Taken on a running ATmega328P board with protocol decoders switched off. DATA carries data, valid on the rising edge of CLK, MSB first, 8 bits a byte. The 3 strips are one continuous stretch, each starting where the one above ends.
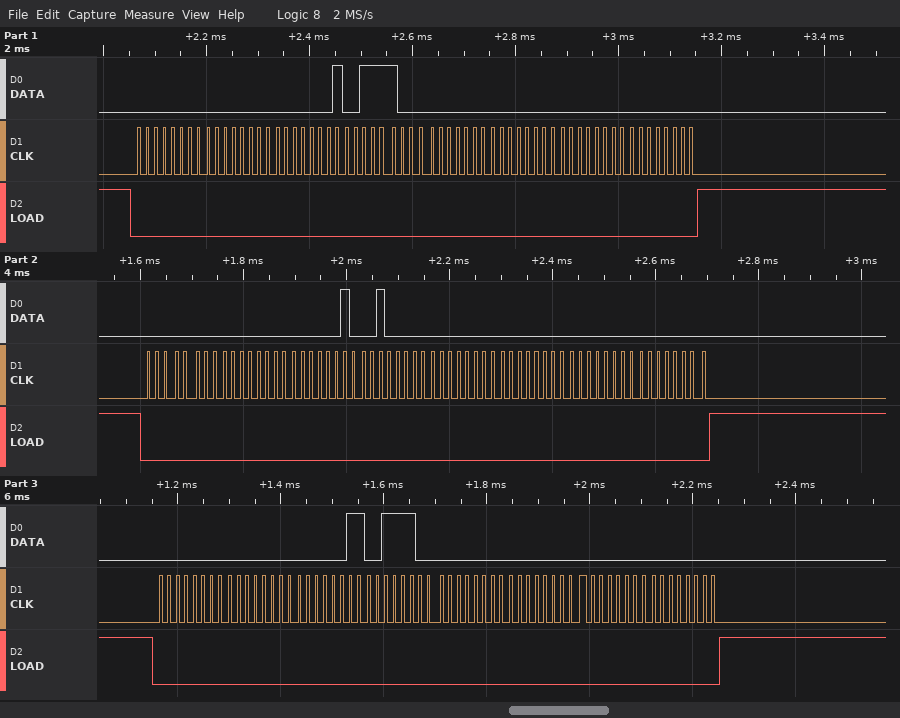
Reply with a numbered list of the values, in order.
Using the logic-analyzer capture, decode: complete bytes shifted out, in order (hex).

1. 0x00 0x00 0x01 0x3C 0x00 0x00 0x00 0x00 0x00 0x00 0x02 0x20 0x00 0x00 0x00 0x00 0x00 0x00 0x03 0x3C 0x00 0x00 0x00 0x00
